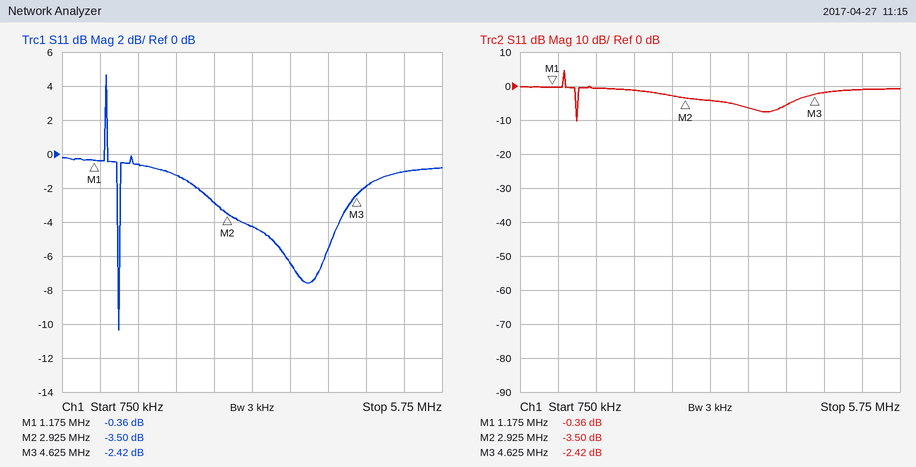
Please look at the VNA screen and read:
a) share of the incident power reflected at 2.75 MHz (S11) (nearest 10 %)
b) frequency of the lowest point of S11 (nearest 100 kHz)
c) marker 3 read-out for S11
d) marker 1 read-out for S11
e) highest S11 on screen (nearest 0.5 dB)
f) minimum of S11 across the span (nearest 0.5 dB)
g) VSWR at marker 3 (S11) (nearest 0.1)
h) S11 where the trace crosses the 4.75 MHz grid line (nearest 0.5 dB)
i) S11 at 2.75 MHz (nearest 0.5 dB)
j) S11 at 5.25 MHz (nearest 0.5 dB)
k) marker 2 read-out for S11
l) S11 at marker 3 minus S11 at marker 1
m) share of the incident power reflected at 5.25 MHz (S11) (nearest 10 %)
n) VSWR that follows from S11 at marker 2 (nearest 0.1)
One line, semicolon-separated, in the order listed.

50 %; 1.5 MHz; -2.42 dB; -0.36 dB; 4.5 dB; -10.5 dB; 7.2; -2.0 dB; -3.0 dB; -1.0 dB; -3.50 dB; -2.06 dB; 80 %; 5.0
